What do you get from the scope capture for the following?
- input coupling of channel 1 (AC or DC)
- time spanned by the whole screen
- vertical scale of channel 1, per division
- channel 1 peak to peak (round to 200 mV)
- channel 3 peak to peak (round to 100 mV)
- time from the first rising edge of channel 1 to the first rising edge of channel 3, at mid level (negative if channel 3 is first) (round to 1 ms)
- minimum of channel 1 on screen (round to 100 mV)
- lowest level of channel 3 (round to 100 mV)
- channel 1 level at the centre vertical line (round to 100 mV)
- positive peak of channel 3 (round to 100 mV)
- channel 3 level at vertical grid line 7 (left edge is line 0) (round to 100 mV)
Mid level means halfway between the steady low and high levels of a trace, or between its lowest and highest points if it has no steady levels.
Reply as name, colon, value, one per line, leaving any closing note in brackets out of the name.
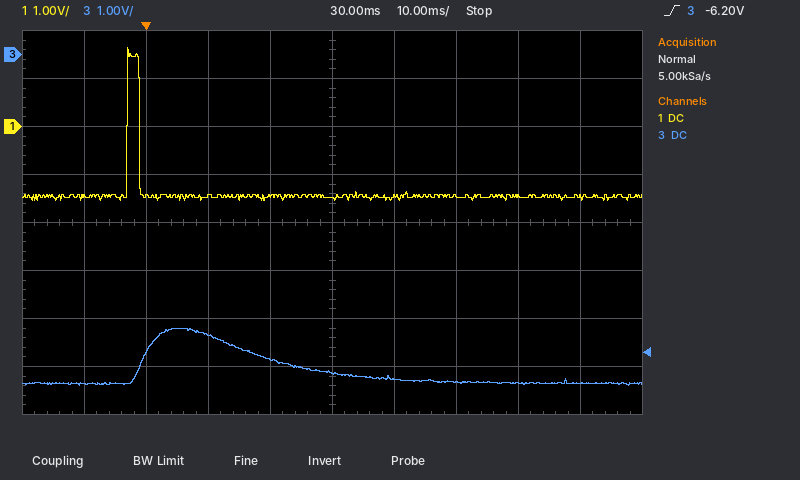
input coupling of channel 1: DC
time spanned by the whole screen: 100 ms
vertical scale of channel 1, per division: 1 V
channel 1 peak to peak: 3.2 V
channel 3 peak to peak: 1.2 V
time from the first rising edge of channel 1 to the first rising edge of channel 3, at mid level (negative if channel 3 is first): +3 ms
minimum of channel 1 on screen: -1.5 V
lowest level of channel 3: -6.9 V
channel 1 level at the centre vertical line: -1.5 V
positive peak of channel 3: -5.7 V
channel 3 level at vertical grid line 7 (left edge is line 0): -6.8 V
